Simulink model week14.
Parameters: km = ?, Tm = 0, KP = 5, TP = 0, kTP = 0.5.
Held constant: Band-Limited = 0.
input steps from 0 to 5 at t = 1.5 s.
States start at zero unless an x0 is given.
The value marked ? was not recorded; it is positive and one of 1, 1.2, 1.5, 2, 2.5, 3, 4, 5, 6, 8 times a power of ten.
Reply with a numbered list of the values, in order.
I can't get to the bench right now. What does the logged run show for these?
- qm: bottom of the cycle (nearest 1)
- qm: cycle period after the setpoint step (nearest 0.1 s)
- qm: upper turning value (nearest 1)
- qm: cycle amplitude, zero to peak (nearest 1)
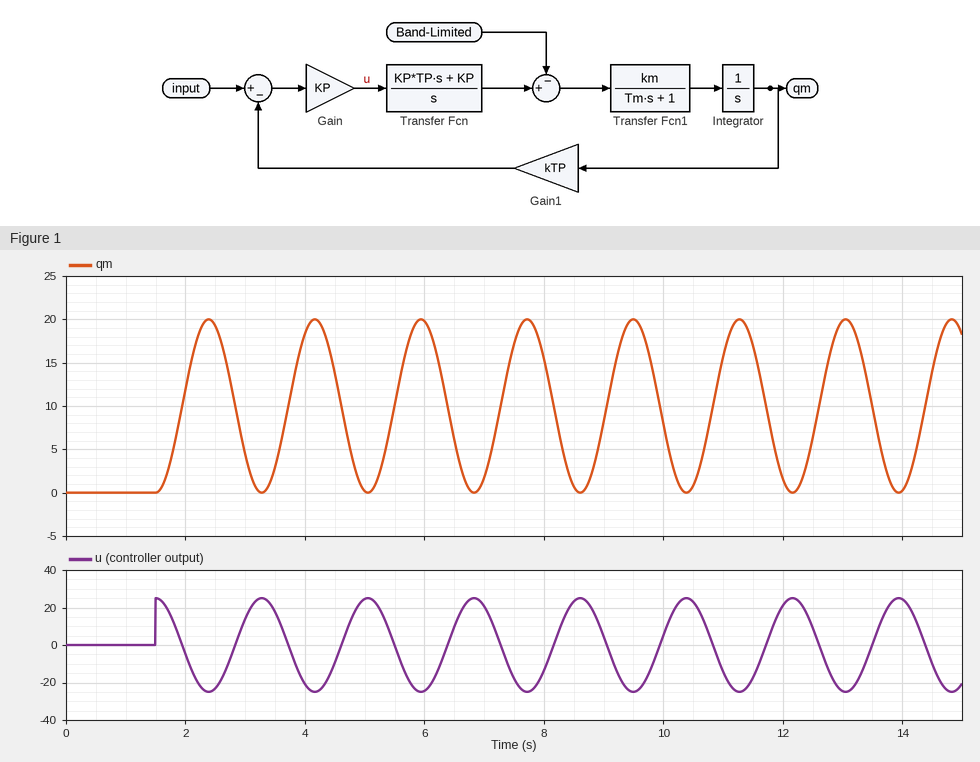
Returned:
1. 0
2. 1.8 s
3. 20
4. 10
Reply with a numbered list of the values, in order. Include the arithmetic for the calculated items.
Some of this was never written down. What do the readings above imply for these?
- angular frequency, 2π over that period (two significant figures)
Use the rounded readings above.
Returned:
1. 2π / 1.8 = 3.5 rad/s
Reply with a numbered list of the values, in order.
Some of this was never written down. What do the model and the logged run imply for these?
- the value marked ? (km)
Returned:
1. 1
